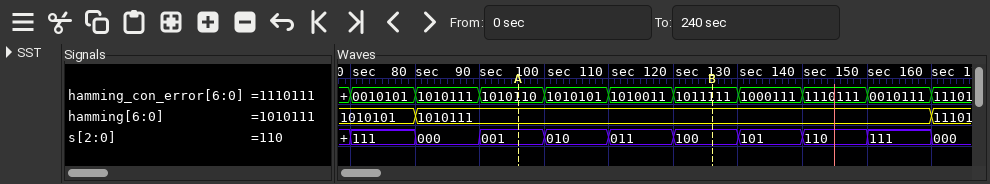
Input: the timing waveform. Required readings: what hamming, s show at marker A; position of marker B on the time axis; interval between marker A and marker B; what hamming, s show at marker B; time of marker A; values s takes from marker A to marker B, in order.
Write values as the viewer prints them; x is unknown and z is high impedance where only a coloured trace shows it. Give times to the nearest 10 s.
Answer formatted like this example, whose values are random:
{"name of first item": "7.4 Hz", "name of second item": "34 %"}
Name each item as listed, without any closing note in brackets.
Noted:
{"what hamming, s show at marker A": "hamming=1010111, s=001", "position of marker B on the time axis": "130 s", "interval between marker A and marker B": "30 s", "what hamming, s show at marker B": "hamming=1010111, s=100", "time of marker A": "100 s", "values s takes from marker A to marker B, in order": "001, 010, 011, 100"}
